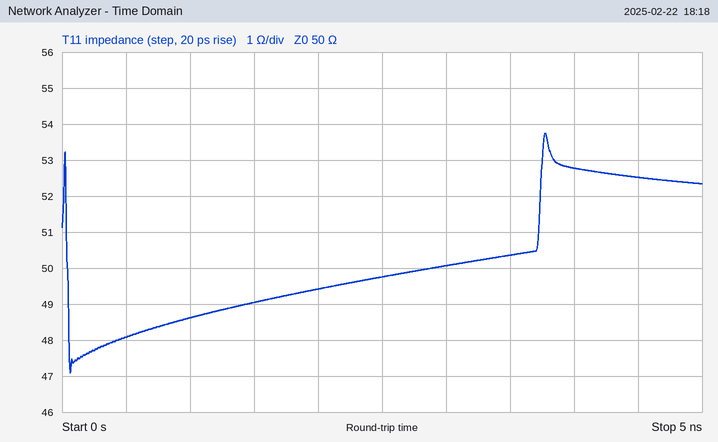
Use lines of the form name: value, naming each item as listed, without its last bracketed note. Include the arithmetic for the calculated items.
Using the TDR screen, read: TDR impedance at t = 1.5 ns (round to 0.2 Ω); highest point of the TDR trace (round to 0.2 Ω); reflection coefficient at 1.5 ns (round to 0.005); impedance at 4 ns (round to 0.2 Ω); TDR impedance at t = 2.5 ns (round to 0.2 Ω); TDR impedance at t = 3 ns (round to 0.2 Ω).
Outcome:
TDR impedance at t = 1.5 ns: 49.0 Ω
highest point of the TDR trace: 53.8 Ω
reflection coefficient at 1.5 ns: (49 − 50)/(49 + 50) ≈ -0.010
impedance at 4 ns: 52.8 Ω
TDR impedance at t = 2.5 ns: 49.8 Ω
TDR impedance at t = 3 ns: 50.0 Ω
